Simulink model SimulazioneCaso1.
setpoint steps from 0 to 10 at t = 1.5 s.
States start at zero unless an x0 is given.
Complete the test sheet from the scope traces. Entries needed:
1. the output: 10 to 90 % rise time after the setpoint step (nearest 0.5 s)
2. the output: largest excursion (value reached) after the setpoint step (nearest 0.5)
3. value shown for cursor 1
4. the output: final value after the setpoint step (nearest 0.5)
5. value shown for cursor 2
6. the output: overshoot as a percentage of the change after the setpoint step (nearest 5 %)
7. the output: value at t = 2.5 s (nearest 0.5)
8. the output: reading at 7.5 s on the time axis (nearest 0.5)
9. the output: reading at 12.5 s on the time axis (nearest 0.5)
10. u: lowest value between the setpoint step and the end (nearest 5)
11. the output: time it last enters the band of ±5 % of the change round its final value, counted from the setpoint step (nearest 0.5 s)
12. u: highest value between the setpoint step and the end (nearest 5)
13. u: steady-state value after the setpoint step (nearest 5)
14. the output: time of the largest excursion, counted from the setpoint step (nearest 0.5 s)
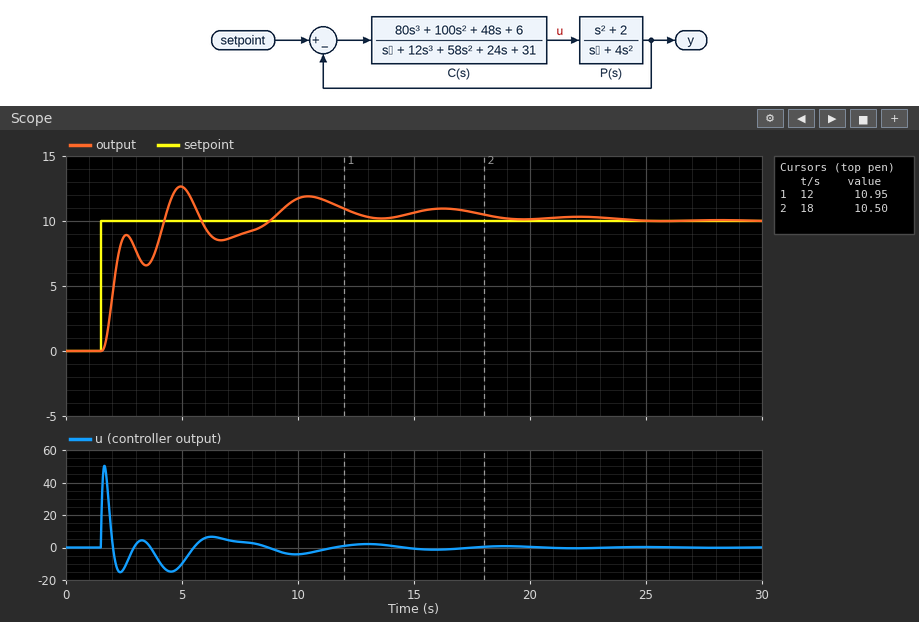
2.5 s
12.5
10.95
10.0
10.50
25 %
9.0
9.0
10.5
-15
16.5 s
50
0
3.5 s
